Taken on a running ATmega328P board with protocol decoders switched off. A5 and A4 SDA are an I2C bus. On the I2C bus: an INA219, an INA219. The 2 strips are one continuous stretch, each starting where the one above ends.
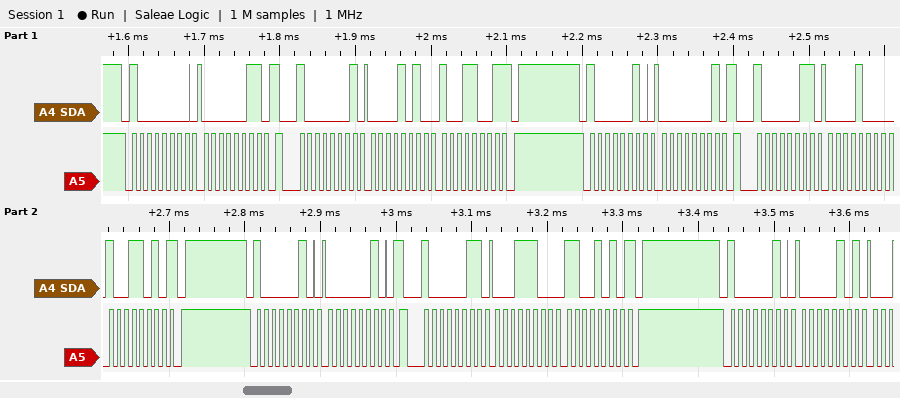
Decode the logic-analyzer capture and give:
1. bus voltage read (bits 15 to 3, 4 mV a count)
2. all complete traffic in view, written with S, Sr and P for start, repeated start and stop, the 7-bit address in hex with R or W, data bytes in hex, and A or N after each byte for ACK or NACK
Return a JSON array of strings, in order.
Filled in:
["3.684 V", "S 40W A 03 A Sr 40R A 0A A 99 N P S 41W A 01 A Sr 41R A 08 A 9A N P S 41W A 02 A Sr 41R A 1C A CA N P S 41W A 05 A"]
